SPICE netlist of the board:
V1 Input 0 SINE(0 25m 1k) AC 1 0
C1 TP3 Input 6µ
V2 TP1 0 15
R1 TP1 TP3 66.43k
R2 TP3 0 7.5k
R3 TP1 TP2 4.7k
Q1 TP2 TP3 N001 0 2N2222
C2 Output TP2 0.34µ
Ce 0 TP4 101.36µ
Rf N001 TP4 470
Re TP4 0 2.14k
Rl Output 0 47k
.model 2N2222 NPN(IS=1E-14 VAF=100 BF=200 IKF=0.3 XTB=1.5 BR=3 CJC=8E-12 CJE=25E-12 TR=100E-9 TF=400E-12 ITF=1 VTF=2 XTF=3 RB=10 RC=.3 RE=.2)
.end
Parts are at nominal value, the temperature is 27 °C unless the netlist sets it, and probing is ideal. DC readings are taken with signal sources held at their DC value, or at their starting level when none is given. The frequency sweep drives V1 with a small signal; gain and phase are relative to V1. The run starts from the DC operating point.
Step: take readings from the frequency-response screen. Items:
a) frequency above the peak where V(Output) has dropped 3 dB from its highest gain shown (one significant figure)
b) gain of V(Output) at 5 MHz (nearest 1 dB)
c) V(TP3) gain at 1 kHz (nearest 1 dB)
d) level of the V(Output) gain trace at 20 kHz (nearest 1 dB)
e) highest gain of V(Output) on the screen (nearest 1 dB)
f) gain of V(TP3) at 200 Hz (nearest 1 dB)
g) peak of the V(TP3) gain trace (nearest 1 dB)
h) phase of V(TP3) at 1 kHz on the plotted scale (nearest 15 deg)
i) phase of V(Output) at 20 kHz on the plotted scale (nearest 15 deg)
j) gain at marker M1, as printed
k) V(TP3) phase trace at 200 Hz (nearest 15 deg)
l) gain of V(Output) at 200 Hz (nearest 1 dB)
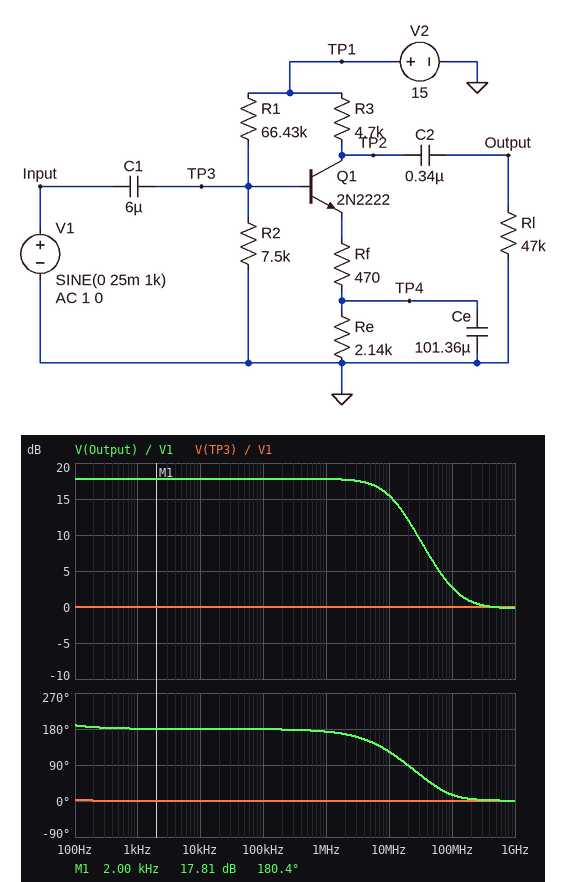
10 MHz
17 dB
0 dB
18 dB
18 dB
0 dB
0 dB
0 deg
180 deg
17.81 dB
0 deg
18 dB
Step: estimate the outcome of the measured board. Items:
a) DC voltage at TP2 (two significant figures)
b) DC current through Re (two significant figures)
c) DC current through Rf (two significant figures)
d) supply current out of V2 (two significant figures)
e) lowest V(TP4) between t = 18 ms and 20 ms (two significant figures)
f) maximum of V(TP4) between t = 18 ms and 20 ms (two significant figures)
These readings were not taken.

13 V
340 µA
340 µA
540 µA
730 mV
730 mV
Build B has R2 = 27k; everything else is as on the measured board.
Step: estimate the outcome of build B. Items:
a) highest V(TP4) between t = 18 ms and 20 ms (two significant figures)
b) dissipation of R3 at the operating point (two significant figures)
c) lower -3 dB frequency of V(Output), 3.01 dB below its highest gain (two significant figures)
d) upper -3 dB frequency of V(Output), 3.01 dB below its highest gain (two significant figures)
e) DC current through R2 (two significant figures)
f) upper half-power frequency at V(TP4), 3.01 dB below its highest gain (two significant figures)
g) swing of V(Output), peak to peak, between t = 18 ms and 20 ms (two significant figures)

2.9 V
8.6 mW
11 Hz
8.8 MHz
160 µA
6.5 Hz
430 mV
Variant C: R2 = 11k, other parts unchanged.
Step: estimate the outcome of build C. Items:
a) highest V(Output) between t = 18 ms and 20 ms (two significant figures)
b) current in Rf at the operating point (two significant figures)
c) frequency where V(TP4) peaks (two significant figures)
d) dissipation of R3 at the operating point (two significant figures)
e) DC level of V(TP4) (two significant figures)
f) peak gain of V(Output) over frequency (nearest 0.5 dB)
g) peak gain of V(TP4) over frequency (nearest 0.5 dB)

210 mV
560 µA
3.3 Hz
1.5 mW
1.2 V
18.5 dB
-7.0 dB
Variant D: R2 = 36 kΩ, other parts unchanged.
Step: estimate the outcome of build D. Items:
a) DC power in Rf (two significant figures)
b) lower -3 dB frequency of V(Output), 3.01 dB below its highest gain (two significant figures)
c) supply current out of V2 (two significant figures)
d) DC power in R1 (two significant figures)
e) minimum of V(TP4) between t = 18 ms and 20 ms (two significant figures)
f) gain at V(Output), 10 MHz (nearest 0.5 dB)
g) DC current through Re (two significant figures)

1.3 mW
11 Hz
1.8 mA
1.5 mW
3.6 V
14.0 dB
1.7 mA
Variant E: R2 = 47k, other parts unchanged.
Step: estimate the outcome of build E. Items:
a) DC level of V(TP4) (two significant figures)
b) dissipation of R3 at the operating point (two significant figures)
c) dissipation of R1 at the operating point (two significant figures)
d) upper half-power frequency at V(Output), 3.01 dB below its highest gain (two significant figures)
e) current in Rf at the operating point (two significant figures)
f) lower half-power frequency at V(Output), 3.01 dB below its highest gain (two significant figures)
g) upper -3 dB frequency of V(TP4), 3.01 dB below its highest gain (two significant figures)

4.3 V
19 mW
1.2 mW
3.7 MHz
2.0 mA
11 Hz
6.0 Hz
